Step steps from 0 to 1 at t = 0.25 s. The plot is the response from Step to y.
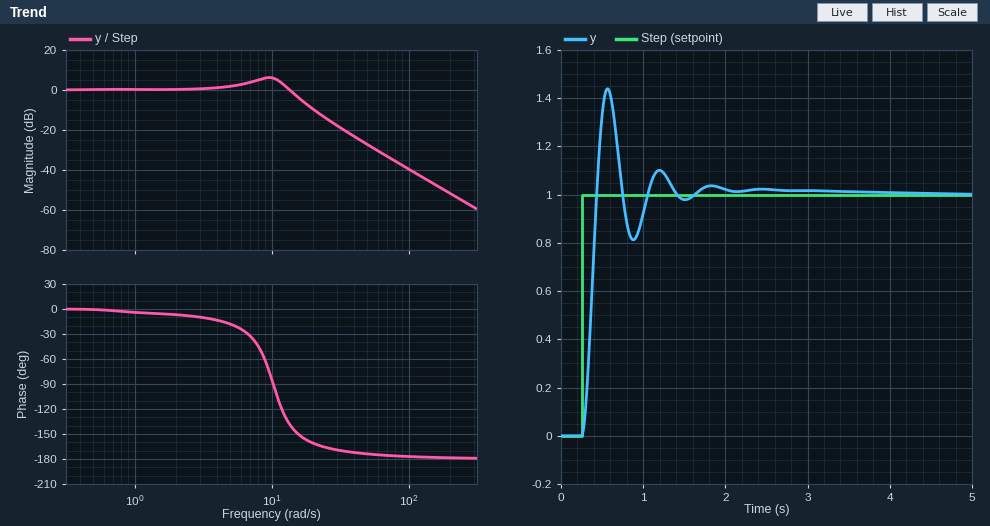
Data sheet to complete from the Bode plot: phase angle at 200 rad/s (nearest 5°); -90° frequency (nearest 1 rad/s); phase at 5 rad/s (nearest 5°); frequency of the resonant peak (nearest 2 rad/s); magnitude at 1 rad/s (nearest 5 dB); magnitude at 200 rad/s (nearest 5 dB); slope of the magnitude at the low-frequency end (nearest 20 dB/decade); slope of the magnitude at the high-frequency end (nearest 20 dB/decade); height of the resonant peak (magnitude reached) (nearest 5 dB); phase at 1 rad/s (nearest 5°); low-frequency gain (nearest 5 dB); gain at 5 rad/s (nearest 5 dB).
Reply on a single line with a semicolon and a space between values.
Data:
-180°; 10 rad/s; -20°; 10 rad/s; 0 dB; -50 dB; 0 dB/decade; -40 dB/decade; 5 dB; -5°; 0 dB; 0 dB
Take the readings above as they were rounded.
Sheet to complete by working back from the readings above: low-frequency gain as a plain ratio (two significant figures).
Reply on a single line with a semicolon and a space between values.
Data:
1.0
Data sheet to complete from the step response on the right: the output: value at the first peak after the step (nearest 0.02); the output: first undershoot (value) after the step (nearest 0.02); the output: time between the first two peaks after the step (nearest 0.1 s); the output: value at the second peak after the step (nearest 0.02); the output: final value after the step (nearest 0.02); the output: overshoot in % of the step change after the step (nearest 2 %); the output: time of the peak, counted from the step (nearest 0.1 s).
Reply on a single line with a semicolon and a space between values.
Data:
1.44; 0.82; 0.6 s; 1.10; 1.00; 44 %; 0.3 s
